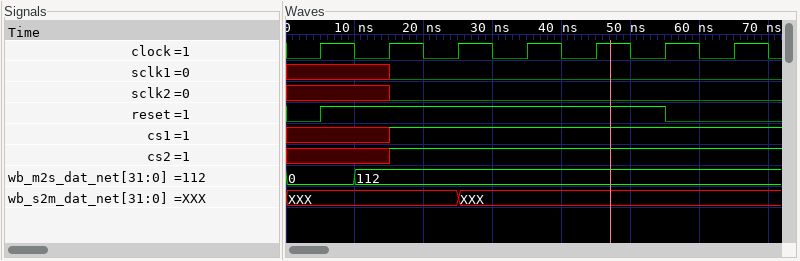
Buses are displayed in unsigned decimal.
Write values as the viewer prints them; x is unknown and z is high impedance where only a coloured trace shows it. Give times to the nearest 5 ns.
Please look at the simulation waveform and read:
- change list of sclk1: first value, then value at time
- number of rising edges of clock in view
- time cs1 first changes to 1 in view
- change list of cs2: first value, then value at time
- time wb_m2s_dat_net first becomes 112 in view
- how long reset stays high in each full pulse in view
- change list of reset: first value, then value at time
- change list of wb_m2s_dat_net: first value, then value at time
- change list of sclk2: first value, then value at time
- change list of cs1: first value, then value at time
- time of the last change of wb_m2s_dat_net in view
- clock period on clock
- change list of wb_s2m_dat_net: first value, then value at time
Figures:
x, 0 at 15 ns
7
15 ns
x, 1 at 15 ns
10 ns
50 ns
0, 1 at 5 ns, 0 at 55 ns
0, 112 at 10 ns
x, 0 at 15 ns
x, 1 at 15 ns
10 ns
10 ns
XXX, XXX at 25 ns
